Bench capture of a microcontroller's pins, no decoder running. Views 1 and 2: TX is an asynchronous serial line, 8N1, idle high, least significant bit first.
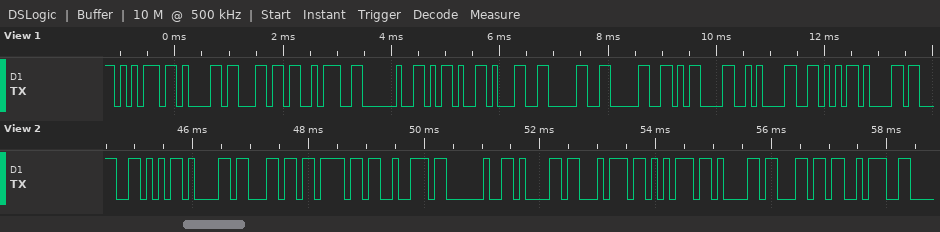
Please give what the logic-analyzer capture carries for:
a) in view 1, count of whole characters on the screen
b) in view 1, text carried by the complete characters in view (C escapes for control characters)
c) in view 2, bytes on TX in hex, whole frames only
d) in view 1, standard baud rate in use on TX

13
"ual: -100\r\nVa"
56 61 6C 6F 72 20 61 74 75 61 6C 3A
9600 baud
